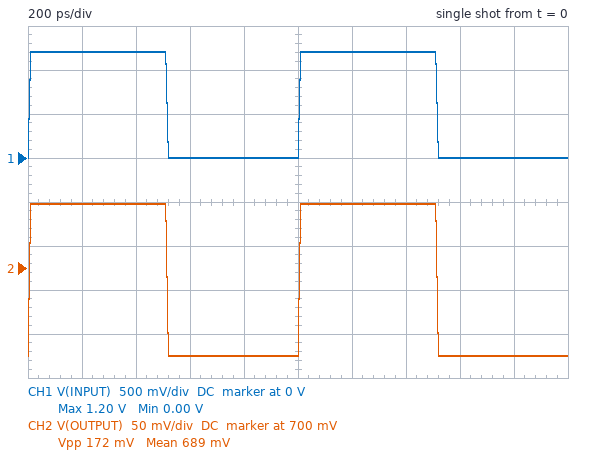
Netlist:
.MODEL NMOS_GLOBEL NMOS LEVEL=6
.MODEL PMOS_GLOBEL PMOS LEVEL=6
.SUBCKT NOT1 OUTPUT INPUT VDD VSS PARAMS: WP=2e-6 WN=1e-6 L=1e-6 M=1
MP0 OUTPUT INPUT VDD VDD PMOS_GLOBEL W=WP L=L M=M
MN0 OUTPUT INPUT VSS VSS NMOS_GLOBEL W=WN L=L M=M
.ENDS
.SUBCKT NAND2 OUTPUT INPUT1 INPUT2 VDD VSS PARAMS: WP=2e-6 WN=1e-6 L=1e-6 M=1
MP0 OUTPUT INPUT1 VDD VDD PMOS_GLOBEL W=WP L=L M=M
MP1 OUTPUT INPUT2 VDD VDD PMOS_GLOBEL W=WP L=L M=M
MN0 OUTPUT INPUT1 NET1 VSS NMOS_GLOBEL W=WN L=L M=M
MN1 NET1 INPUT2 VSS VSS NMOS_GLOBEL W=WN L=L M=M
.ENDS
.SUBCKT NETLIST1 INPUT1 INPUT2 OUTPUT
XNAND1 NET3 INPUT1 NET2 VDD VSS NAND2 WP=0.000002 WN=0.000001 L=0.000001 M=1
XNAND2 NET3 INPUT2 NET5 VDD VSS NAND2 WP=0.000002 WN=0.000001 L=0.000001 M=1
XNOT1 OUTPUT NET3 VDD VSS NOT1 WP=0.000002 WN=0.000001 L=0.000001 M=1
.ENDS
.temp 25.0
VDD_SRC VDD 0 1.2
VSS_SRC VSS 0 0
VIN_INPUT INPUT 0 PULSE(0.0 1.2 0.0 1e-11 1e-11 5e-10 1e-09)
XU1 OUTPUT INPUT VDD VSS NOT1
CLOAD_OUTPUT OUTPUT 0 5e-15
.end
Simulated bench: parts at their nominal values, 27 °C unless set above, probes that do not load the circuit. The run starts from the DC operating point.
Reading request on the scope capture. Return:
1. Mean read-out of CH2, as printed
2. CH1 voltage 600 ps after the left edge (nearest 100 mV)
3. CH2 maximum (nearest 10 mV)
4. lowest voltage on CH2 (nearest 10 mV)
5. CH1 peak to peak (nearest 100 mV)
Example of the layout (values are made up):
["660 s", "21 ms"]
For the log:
["689 mV", "0 V", "770 mV", "600 mV", "1.2 V"]
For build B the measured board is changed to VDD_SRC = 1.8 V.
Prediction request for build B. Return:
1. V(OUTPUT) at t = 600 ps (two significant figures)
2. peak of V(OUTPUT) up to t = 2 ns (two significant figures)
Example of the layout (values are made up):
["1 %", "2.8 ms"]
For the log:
["1.8 V", "2.0 V"]
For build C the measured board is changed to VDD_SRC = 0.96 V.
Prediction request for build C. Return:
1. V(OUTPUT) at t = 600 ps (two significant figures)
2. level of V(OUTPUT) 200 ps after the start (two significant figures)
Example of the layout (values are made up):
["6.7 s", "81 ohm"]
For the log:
["480 mV", "650 mV"]
